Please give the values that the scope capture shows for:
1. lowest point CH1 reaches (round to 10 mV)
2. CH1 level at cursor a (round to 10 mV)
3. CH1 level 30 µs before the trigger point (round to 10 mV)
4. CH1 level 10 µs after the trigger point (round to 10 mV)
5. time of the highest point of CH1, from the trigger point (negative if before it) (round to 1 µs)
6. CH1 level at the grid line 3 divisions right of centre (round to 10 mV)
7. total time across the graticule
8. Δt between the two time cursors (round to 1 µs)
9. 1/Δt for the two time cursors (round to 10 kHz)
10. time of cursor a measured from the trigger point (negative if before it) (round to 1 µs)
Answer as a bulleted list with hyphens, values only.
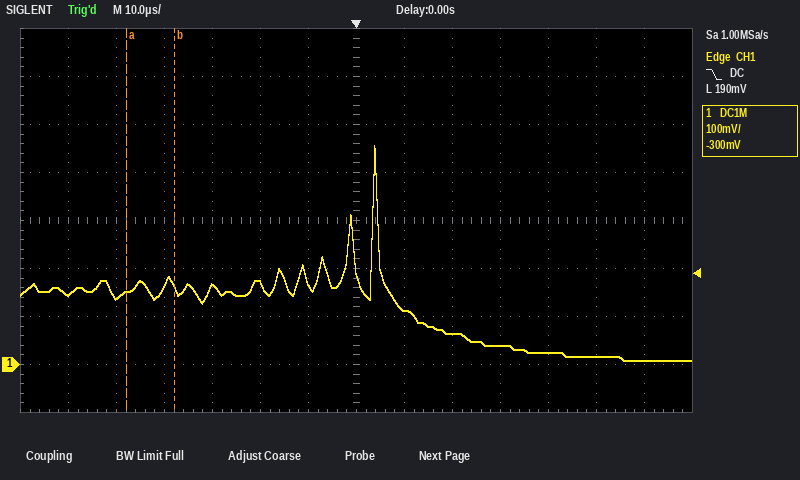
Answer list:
- 10 mV
- 150 mV
- 160 mV
- 110 mV
- +4 µs
- 40 mV
- 140 µs
- 10 µs
- 100 kHz
- -48 µs
